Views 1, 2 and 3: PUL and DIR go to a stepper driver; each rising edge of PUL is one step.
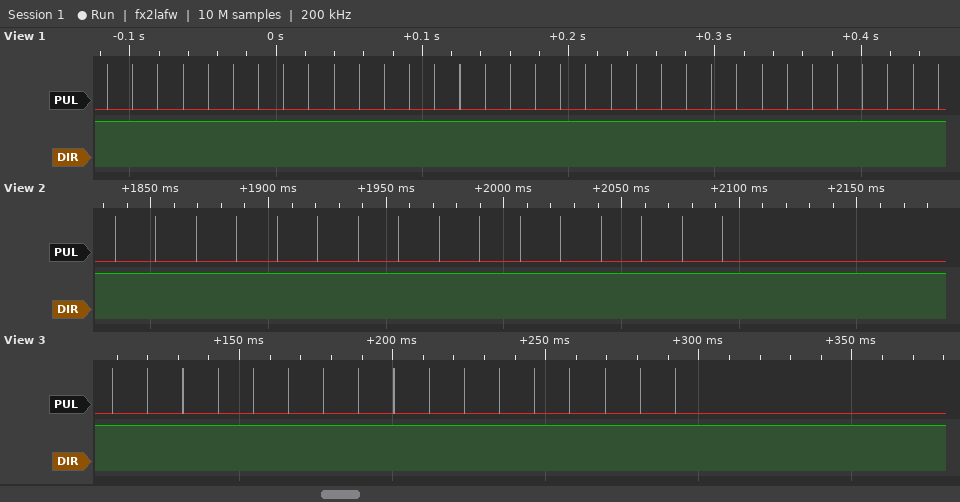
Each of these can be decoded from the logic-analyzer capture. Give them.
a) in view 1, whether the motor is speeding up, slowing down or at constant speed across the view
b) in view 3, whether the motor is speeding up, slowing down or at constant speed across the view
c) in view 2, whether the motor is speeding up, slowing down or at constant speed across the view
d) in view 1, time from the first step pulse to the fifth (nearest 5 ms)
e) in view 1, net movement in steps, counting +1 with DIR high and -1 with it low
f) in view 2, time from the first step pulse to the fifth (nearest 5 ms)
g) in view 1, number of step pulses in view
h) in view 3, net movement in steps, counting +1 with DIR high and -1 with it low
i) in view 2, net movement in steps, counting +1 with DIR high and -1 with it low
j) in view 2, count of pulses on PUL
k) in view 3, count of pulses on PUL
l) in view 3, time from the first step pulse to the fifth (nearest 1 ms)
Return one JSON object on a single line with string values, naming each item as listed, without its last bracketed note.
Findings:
{"in view 1, whether the motor is speeding up, slowing down or at constant speed across the view": "constant speed", "in view 3, whether the motor is speeding up, slowing down or at constant speed across the view": "constant speed", "in view 2, whether the motor is speeding up, slowing down or at constant speed across the view": "constant speed", "in view 1, time from the first step pulse to the fifth": "70 ms", "in view 1, net movement in steps, counting +1 with DIR high and -1 with it low": "+34", "in view 2, time from the first step pulse to the fifth": "70 ms", "in view 1, number of step pulses in view": "34", "in view 3, net movement in steps, counting +1 with DIR high and -1 with it low": "+17", "in view 2, net movement in steps, counting +1 with DIR high and -1 with it low": "+16", "in view 2, count of pulses on PUL": "16", "in view 3, count of pulses on PUL": "17", "in view 3, time from the first step pulse to the fifth": "46 ms"}
